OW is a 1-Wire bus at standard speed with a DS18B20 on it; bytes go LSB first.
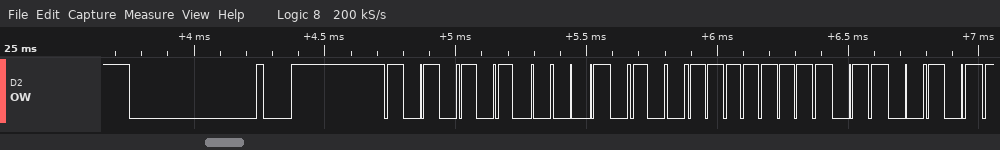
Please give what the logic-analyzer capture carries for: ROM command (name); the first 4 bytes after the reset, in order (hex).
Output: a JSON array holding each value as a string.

["Match ROM", "55 28 FF A6"]
